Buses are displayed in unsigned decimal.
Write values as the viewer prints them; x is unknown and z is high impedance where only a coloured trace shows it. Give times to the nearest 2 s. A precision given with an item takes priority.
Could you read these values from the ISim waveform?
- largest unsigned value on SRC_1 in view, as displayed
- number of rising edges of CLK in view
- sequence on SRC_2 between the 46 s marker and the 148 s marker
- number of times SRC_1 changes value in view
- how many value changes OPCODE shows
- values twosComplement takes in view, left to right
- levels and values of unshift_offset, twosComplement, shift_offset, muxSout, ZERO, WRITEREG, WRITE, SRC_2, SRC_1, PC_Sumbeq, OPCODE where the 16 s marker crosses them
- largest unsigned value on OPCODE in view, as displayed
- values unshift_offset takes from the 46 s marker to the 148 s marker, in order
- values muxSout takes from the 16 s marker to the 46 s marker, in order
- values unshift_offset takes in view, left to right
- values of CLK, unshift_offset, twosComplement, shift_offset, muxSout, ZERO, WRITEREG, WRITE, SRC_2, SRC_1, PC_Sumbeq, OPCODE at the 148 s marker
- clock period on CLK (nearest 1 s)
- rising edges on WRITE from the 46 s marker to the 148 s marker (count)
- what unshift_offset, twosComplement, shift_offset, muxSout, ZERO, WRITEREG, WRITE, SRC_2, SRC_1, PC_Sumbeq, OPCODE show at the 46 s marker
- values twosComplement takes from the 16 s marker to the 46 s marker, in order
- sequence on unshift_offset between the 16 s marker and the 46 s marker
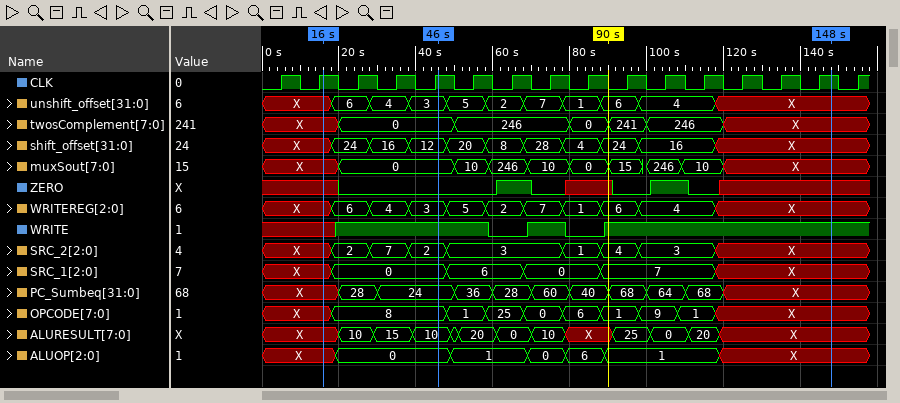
7
16
2, 3, 1, 4, 3, X
5
9
X, 0, 246, 0, 241, 246, X
unshift_offset=X, twosComplement=X, shift_offset=X, muxSout=X, ZERO=x, WRITEREG=X, WRITE=x, SRC_2=X, SRC_1=X, PC_Sumbeq=X, OPCODE=X
25
3, 5, 2, 7, 1, 6, 4, X
X, 0
X, 6, 4, 3, 5, 2, 7, 1, 6, 4, X
CLK=1, unshift_offset=X, twosComplement=X, shift_offset=X, muxSout=X, ZERO=x, WRITEREG=X, WRITE=1, SRC_2=X, SRC_1=X, PC_Sumbeq=X, OPCODE=X
10 s
2
unshift_offset=3, twosComplement=0, shift_offset=12, muxSout=0, ZERO=0, WRITEREG=3, WRITE=1, SRC_2=2, SRC_1=0, PC_Sumbeq=24, OPCODE=8
X, 0
X, 6, 4, 3
